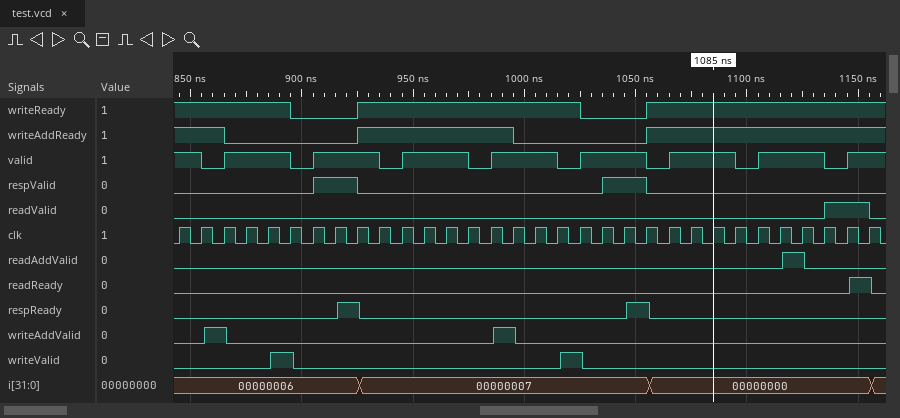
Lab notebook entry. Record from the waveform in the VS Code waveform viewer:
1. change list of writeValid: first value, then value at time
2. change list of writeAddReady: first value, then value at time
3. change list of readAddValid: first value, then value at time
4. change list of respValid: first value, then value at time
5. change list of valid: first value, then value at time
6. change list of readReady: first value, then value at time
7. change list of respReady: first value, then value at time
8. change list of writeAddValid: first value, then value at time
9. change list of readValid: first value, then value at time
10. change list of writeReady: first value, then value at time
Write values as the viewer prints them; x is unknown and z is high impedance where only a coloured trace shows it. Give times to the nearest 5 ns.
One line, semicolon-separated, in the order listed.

0, 1 at 885 ns, 0 at 895 ns, 1 at 1015 ns, 0 at 1025 ns; 1, 0 at 865 ns, 1 at 925 ns, 0 at 995 ns, 1 at 1055 ns; 0, 1 at 1115 ns, 0 at 1125 ns; 0, 1 at 905 ns, 0 at 925 ns, 1 at 1035 ns, 0 at 1055 ns; 1, 0 at 855 ns, 1 at 865 ns, 0 at 895 ns, 1 at 905 ns, 0 at 935 ns, 1 at 945 ns, 0 at 975 ns, 1 at 985 ns, 0 at 1015 ns, 1 at 1025 ns, 0 at 1055 ns, 1 at 1065 ns, 0 at 1095 ns, 1 at 1105 ns, 0 at 1135 ns, 1 at 1145 ns; 0, 1 at 1145 ns, 0 at 1155 ns; 0, 1 at 915 ns, 0 at 925 ns, 1 at 1045 ns, 0 at 1055 ns; 0, 1 at 855 ns, 0 at 865 ns, 1 at 985 ns, 0 at 995 ns; 0, 1 at 1135 ns, 0 at 1155 ns; 1, 0 at 895 ns, 1 at 925 ns, 0 at 1025 ns, 1 at 1055 ns
